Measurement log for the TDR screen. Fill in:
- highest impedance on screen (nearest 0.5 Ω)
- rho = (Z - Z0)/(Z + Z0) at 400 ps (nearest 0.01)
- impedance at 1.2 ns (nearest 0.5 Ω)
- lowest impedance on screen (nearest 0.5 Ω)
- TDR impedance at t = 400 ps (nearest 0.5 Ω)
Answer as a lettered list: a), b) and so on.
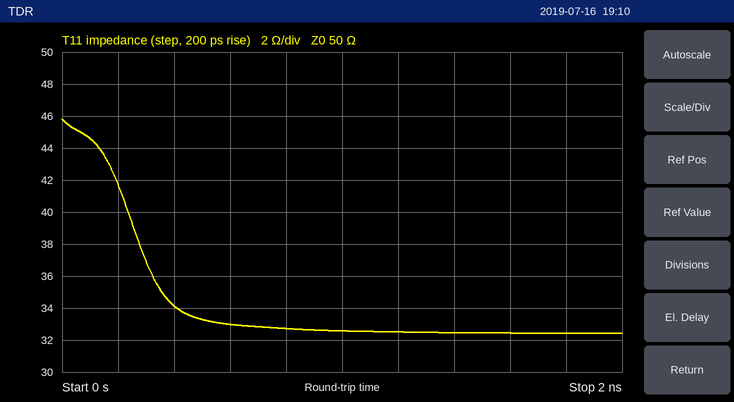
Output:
a) 46.0 Ω
b) -0.19
c) 32.5 Ω
d) 32.5 Ω
e) 34.0 Ω
